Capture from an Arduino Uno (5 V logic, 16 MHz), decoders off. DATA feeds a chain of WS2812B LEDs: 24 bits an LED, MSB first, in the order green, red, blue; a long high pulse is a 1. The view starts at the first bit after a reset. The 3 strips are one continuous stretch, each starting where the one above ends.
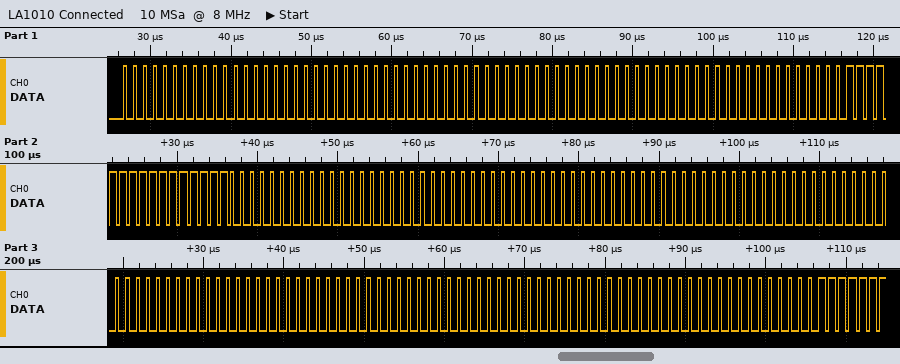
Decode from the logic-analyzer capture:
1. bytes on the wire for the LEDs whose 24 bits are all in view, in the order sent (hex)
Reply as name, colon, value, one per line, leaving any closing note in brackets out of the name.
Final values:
bytes on the wire for the LEDs whose 24 bits are all in view, in the order sent: 00 00 00 00 00 00 00 00 00 FF FF 00 00 00 00 00 00 00 00 00 00 00 00 00 00 00 00
